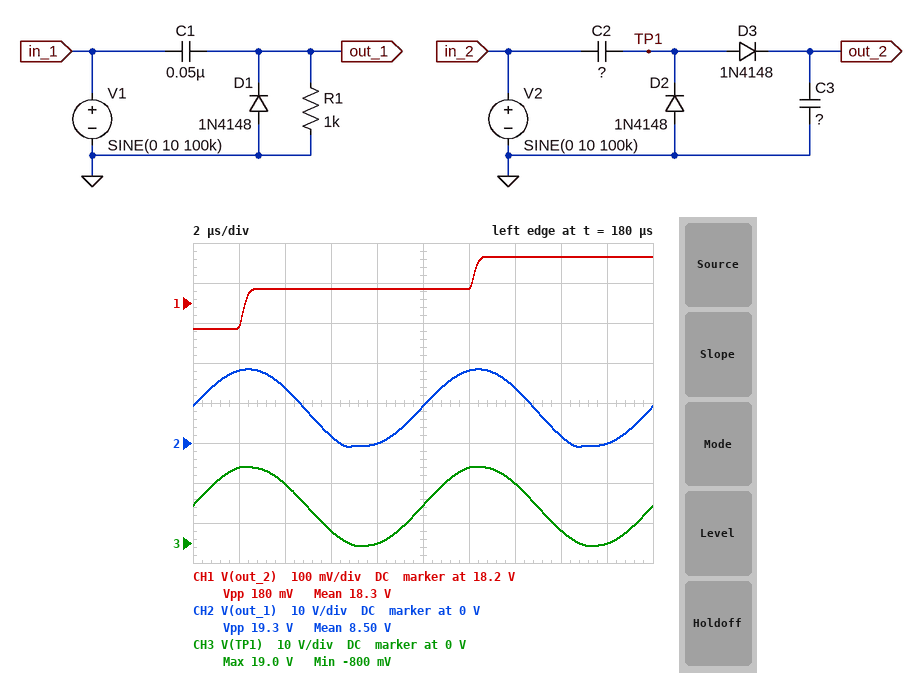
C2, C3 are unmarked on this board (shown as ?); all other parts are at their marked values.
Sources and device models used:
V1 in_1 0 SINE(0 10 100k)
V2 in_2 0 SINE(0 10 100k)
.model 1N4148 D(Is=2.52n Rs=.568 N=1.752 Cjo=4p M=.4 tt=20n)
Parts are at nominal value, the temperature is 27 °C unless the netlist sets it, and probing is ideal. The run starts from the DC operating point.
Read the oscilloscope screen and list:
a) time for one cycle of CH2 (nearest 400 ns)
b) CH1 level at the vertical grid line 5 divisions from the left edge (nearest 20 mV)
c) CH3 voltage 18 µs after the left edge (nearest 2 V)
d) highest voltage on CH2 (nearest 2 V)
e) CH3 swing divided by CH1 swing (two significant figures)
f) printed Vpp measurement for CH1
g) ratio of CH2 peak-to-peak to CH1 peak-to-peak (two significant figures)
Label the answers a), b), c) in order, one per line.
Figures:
a) 10.0 µs
b) 18.24 V
c) 0 V
d) 18 V
e) 110
f) 180 mV
g) 110
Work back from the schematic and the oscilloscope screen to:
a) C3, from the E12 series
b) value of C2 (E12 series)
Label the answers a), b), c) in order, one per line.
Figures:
a) 120 nF
b) 27 nF
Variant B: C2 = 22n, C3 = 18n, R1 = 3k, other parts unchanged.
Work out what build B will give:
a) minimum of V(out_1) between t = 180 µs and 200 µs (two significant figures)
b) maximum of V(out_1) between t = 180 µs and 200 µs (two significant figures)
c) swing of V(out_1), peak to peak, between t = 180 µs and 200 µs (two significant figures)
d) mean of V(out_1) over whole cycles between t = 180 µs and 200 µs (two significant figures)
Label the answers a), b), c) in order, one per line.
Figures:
a) -820 mV
b) 19 V
c) 20 V
d) 9.0 V
